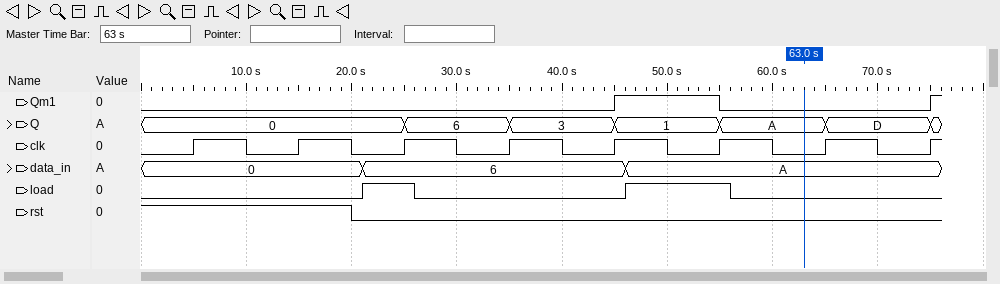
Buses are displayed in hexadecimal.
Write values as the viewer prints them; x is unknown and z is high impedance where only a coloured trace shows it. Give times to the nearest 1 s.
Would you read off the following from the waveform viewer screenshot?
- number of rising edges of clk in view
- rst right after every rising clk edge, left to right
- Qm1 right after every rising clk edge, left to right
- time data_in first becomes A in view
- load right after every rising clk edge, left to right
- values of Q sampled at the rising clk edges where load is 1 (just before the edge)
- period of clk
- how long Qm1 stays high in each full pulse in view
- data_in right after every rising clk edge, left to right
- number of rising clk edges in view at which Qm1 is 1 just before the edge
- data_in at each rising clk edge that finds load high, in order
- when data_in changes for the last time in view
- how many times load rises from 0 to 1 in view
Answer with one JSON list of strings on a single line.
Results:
["8", "1 1 0 0 0 0 0 0", "0 0 0 0 1 0 0 1", "46 s", "0 0 1 0 0 1 0 0", "0, 1", "10 s", "10 s", "0, 0, 6, 6, 6, A, A, A", "1", "6, A", "46 s", "2"]
